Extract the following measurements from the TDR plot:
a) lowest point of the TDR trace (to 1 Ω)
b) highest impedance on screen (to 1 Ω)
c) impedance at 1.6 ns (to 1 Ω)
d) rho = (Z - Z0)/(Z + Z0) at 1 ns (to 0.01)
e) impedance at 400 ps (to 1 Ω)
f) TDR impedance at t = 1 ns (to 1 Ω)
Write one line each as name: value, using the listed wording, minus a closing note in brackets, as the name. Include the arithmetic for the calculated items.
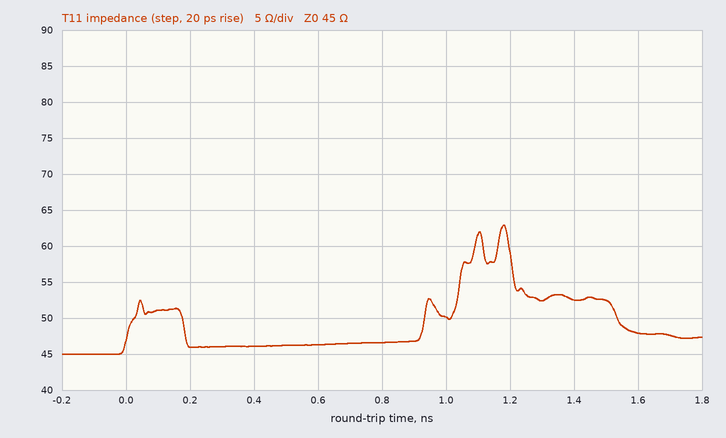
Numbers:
lowest point of the TDR trace: 45 Ω
highest impedance on screen: 63 Ω
impedance at 1.6 ns: 48 Ω
rho = (Z - Z0)/(Z + Z0) at 1 ns: (50 − 45)/(50 + 45) ≈ +0.05
impedance at 400 ps: 46 Ω
TDR impedance at t = 1 ns: 50 Ω
